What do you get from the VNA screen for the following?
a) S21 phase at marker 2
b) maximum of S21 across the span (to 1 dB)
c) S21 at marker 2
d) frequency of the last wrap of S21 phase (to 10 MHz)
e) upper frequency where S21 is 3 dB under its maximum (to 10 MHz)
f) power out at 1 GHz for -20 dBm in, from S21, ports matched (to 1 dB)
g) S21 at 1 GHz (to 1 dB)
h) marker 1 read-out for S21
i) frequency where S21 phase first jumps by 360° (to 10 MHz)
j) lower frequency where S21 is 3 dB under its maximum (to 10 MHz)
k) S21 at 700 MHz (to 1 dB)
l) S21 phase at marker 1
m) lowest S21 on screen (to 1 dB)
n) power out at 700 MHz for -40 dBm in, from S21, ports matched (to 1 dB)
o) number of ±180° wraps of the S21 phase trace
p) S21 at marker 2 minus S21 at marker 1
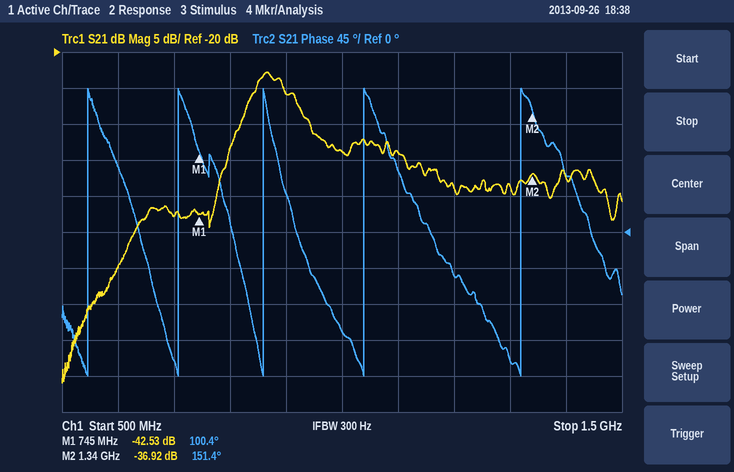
151.4°
-23 dB
-36.92 dB
1.32 GHz
900 MHz
-54 dBm
-34 dB
-42.53 dB
550 MHz
840 MHz
-43 dB
100.4°
-66 dB
-83 dBm
5
5.61 dB
